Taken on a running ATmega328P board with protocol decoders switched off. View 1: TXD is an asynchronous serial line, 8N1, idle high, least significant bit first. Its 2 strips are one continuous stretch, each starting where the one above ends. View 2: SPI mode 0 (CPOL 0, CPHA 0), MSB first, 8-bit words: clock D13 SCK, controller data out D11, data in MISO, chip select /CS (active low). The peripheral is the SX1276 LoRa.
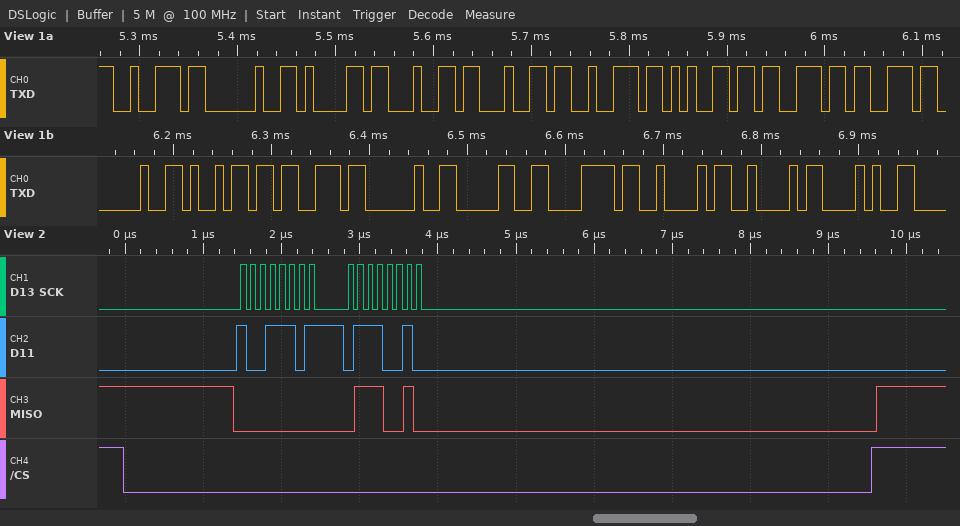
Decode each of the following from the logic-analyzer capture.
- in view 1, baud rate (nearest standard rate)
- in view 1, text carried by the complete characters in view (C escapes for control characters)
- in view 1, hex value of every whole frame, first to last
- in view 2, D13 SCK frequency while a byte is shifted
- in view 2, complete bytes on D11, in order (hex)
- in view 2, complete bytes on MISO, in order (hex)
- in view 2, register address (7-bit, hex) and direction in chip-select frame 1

115200 baud
"r address is 0xBB("
72 20 61 64 64 72 65 73 73 20 69 73 20 30 78 42 42 28
8 MHz
9D 72
00 72
0x1D write
